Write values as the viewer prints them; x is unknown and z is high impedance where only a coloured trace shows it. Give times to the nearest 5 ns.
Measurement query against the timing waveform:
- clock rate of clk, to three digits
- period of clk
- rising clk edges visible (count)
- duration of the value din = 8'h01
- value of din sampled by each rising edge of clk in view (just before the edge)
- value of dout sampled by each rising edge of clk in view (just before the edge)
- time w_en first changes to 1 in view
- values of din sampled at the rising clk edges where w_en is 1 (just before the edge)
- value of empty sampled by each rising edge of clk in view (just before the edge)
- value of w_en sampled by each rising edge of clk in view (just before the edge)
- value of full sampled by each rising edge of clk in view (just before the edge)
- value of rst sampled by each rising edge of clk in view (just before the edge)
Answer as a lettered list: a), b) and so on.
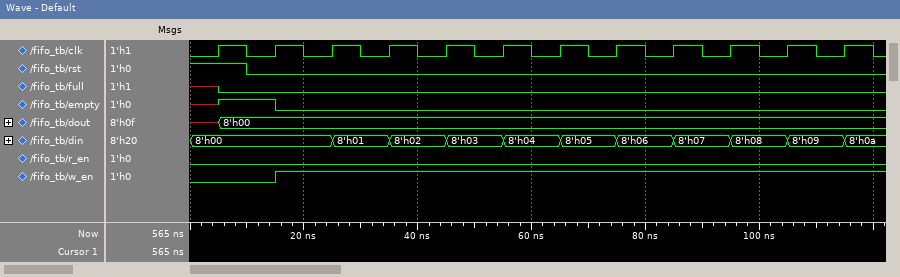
a) 100 MHz
b) 10 ns
c) 12
d) 10 ns
e) 8'h00, 8'h00, 8'h00, 8'h01, 8'h02, 8'h03, 8'h04, 8'h05, 8'h06, 8'h07, 8'h08, 8'h09
f) x, 8'h00, 8'h00, 8'h00, 8'h00, 8'h00, 8'h00, 8'h00, 8'h00, 8'h00, 8'h00, 8'h00
g) 15 ns
h) 8'h00, 8'h01, 8'h02, 8'h03, 8'h04, 8'h05, 8'h06, 8'h07, 8'h08, 8'h09
i) x 1 0 0 0 0 0 0 0 0 0 0
j) 0 0 1 1 1 1 1 1 1 1 1 1
k) x 0 0 0 0 0 0 0 0 0 0 0
l) 1 0 0 0 0 0 0 0 0 0 0 0
